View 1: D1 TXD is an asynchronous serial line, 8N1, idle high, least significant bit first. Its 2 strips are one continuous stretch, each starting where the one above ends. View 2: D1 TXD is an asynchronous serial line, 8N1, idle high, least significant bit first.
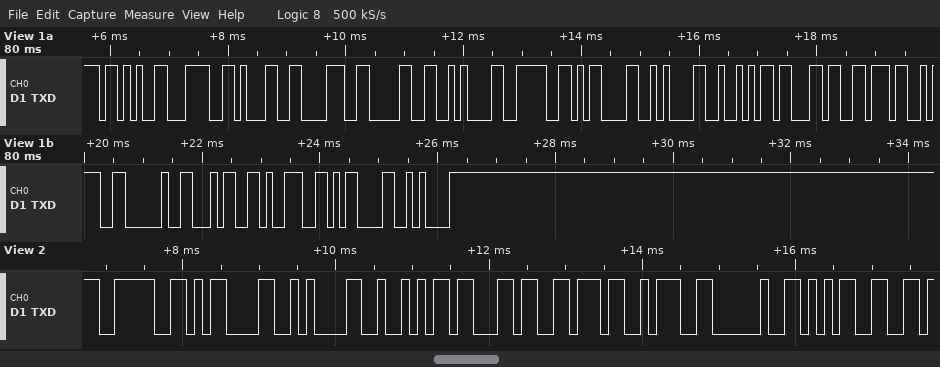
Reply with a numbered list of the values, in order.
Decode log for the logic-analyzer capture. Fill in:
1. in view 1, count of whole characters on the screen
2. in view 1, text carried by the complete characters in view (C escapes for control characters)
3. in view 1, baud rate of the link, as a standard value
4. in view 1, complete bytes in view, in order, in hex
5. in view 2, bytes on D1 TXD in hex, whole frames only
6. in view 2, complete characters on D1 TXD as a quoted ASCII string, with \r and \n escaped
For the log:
1. 18
2. "+<180\n>\r\nRcv: 49\r\n"
3. 9600 baud
4. 2B 3C 31 38 30 0A 3E 0D 0A 52 63 76 3A 20 34 39 0D 0A
5. 3E 0D 0A 52 63 76 3A 20 35
6. ">\r\nRcv: 5"
